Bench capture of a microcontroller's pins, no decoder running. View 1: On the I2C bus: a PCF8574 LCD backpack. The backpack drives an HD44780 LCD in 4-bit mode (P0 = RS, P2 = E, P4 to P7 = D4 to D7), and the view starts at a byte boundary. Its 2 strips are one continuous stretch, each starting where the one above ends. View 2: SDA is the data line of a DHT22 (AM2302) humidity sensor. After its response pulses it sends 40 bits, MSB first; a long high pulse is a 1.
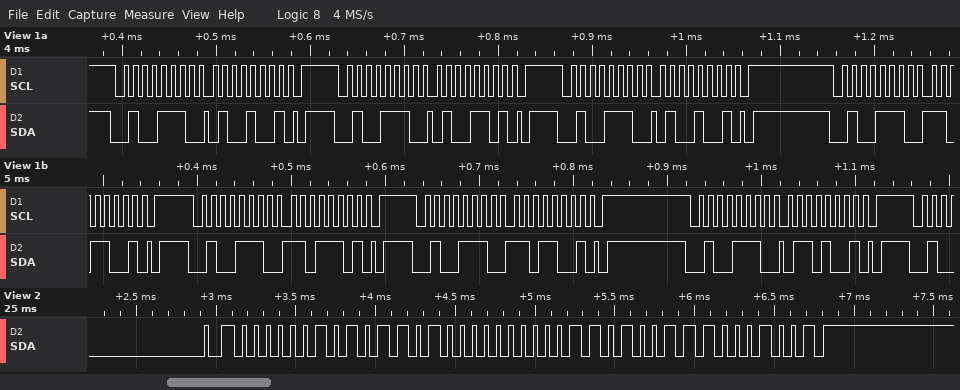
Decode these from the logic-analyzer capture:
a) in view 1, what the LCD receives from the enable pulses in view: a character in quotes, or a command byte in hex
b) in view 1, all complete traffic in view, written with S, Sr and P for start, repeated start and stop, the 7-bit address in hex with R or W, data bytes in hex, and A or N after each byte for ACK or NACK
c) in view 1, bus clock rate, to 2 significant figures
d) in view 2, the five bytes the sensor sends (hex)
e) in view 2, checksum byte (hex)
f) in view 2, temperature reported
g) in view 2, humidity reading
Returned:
'M'
S 27W A 49 A P S 27W A 4D A P S 27W A 49 A P S 27W A D9 A P S 27W A DD A P S 27W A D9 A P S 27W A 69 A P
100 kHz
02 B4 00 D3 89
0x89
21.1 °C
69.2 %
